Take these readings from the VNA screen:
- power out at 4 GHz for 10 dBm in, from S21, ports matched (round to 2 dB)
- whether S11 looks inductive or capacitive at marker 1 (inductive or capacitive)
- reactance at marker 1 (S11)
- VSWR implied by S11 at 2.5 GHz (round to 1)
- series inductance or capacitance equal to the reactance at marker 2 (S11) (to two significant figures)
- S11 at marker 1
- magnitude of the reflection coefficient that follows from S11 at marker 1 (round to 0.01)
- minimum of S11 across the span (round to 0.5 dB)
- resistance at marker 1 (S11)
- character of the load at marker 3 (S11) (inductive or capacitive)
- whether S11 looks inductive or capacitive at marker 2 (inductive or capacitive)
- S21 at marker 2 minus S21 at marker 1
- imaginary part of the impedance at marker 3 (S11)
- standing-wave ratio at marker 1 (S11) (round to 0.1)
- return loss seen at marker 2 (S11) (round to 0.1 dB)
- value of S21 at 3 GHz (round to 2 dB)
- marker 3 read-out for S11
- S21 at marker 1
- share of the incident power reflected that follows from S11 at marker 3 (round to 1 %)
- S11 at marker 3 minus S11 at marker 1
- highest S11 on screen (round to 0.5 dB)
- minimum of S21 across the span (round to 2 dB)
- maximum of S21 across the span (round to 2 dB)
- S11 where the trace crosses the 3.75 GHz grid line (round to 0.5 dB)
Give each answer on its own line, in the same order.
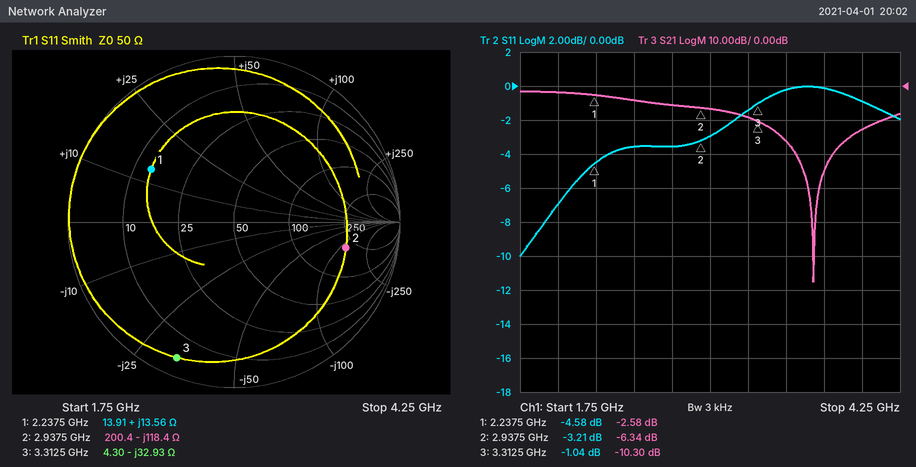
-2 dBm
inductive
+13.56 Ω
5
460 fF
-4.58 dB
0.59
-10.0 dB
13.91 Ω
capacitive
capacitive
-3.76 dB
-32.93 Ω
3.9
3.2 dB
-6 dB
-1.04 dB
-2.58 dB
79 %
3.54 dB
0.0 dB
-58 dB
-2 dB
0.0 dB
